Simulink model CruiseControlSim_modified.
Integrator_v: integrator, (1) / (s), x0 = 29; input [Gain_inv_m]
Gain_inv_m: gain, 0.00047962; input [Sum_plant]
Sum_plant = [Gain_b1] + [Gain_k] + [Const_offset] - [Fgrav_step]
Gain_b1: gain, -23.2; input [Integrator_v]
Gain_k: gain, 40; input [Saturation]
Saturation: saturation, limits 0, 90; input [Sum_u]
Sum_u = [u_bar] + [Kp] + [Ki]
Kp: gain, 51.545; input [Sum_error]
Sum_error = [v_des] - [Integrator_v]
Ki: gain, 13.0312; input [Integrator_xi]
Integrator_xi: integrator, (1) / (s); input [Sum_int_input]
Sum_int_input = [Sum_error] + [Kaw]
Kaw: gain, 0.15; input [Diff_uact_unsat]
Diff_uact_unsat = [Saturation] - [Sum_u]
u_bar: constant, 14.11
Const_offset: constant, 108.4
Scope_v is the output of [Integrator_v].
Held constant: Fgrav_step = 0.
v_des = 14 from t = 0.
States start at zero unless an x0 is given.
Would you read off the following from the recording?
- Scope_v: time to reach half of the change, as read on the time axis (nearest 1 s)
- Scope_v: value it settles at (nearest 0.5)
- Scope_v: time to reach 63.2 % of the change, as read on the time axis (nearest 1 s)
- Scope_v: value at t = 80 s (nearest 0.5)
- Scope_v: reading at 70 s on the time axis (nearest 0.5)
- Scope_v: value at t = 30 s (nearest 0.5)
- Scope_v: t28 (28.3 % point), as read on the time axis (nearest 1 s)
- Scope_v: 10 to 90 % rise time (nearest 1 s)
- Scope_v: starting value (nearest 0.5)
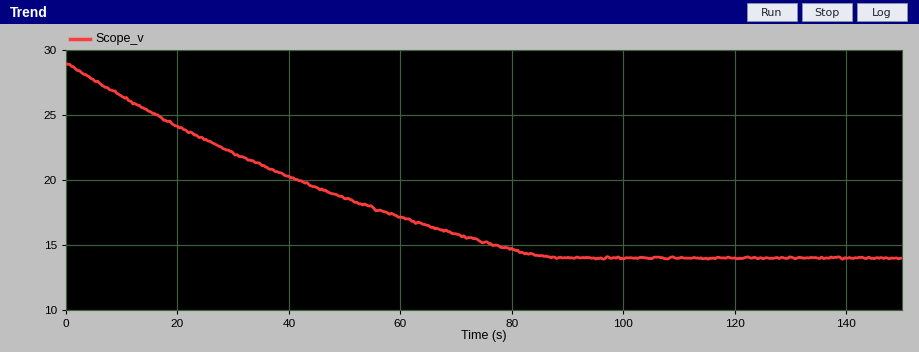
33 s
14.0
44 s
14.5
16.0
22.0
17 s
67 s
29.0
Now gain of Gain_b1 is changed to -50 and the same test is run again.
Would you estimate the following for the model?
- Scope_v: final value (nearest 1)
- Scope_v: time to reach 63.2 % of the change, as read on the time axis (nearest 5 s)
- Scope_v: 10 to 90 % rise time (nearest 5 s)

14
20 s
25 s
